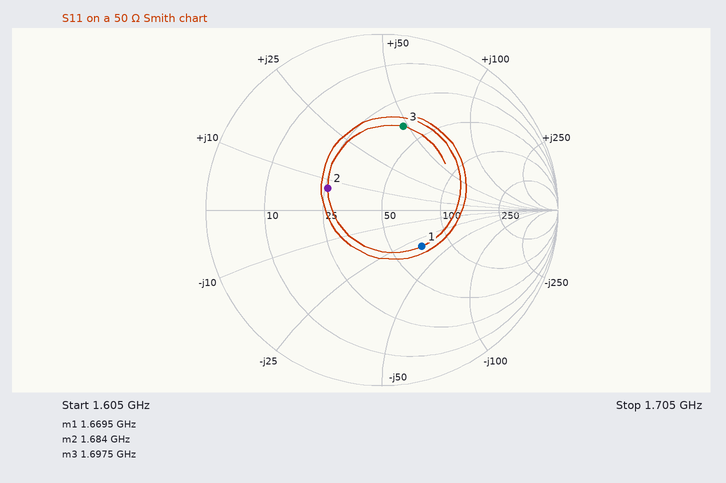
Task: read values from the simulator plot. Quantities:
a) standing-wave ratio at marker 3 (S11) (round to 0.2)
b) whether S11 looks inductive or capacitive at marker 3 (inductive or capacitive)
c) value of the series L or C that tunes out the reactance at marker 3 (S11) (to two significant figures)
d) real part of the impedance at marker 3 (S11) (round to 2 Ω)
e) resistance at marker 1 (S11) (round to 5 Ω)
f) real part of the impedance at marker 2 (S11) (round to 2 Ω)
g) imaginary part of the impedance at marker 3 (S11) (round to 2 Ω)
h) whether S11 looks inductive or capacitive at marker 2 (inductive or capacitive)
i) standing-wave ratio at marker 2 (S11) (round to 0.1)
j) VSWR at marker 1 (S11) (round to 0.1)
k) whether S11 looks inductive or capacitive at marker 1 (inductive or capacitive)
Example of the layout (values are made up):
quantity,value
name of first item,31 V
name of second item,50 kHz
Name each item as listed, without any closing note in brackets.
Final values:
quantity,value
standing-wave ratio at marker 3 (S11),3.0
whether S11 looks inductive or capacitive at marker 3,inductive
value of the series L or C that tunes out the reactance at marker 3 (S11),2.0 pF
real part of the impedance at marker 3 (S11),38 Ω
resistance at marker 1 (S11),70 Ω
real part of the impedance at marker 2 (S11),26 Ω
imaginary part of the impedance at marker 3 (S11),+48 Ω
whether S11 looks inductive or capacitive at marker 2,inductive
standing-wave ratio at marker 2 (S11),2.0
VSWR at marker 1 (S11),1.9
whether S11 looks inductive or capacitive at marker 1,capacitive
